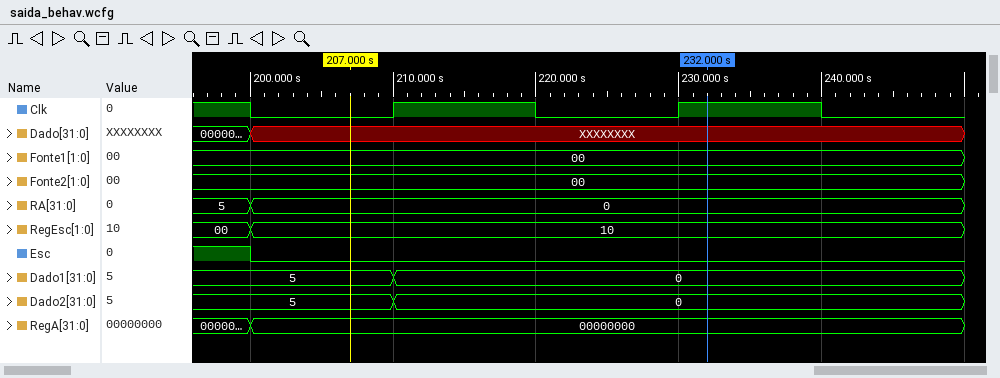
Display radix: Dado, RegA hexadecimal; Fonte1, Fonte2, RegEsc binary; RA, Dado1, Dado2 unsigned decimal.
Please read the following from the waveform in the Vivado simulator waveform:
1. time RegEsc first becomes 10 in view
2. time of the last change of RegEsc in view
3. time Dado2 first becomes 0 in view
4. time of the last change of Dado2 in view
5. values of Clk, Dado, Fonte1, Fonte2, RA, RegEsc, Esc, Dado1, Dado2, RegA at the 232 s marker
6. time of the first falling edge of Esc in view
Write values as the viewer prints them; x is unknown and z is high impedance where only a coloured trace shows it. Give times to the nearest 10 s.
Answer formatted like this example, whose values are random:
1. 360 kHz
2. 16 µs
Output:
1. 200 s
2. 200 s
3. 210 s
4. 210 s
5. Clk=1, Dado=XXXXXXXX, Fonte1=00, Fonte2=00, RA=0, RegEsc=10, Esc=0, Dado1=0, Dado2=0, RegA=00000000
6. 200 s
